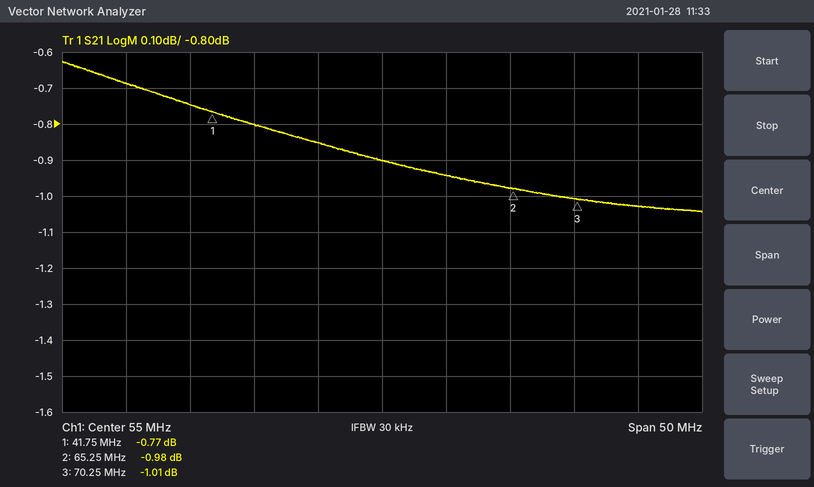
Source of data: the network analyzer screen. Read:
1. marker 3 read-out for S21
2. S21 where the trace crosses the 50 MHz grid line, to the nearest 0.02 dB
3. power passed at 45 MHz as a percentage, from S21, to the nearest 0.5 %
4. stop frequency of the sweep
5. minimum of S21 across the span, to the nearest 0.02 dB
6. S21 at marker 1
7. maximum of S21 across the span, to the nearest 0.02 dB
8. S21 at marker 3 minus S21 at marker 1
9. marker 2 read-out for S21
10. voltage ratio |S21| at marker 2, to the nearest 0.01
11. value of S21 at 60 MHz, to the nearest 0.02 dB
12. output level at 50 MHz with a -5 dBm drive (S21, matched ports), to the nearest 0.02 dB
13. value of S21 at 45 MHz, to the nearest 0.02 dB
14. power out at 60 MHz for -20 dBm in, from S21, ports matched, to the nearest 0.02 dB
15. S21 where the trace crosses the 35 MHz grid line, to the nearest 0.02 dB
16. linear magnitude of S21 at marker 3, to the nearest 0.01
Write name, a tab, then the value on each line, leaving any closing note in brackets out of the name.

marker 3 read-out for S21	-1.01 dB
S21 where the trace crosses the 50 MHz grid line, to the nearest 0.02 dB	-0.86 dB
power passed at 45 MHz as a percentage, from S21, to the nearest 0.5 %	83.0 %
stop frequency of the sweep	80 MHz
minimum of S21 across the span, to the nearest 0.02 dB	-1.04 dB
S21 at marker 1	-0.77 dB
maximum of S21 across the span, to the nearest 0.02 dB	-0.62 dB
S21 at marker 3 minus S21 at marker 1	-0.24 dB
marker 2 read-out for S21	-0.98 dB
voltage ratio |S21| at marker 2, to the nearest 0.01	0.89
value of S21 at 60 MHz, to the nearest 0.02 dB	-0.94 dB
output level at 50 MHz with a -5 dBm drive (S21, matched ports), to the nearest 0.02 dB	-5.86 dBm
value of S21 at 45 MHz, to the nearest 0.02 dB	-0.80 dB
power out at 60 MHz for -20 dBm in, from S21, ports matched, to the nearest 0.02 dB	-20.94 dBm
S21 where the trace crosses the 35 MHz grid line, to the nearest 0.02 dB	-0.68 dB
linear magnitude of S21 at marker 3, to the nearest 0.01	0.89
